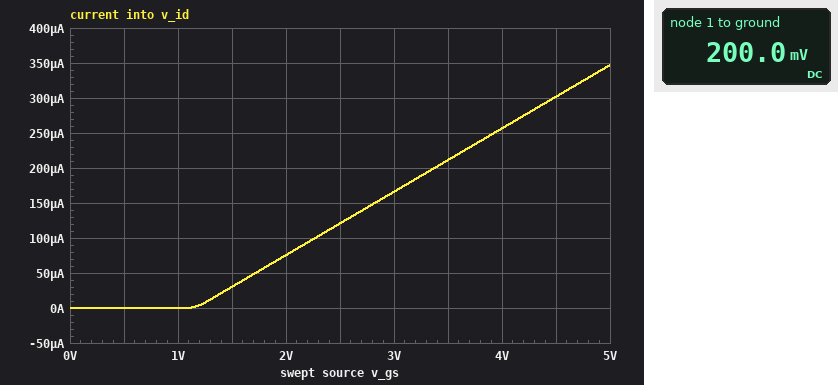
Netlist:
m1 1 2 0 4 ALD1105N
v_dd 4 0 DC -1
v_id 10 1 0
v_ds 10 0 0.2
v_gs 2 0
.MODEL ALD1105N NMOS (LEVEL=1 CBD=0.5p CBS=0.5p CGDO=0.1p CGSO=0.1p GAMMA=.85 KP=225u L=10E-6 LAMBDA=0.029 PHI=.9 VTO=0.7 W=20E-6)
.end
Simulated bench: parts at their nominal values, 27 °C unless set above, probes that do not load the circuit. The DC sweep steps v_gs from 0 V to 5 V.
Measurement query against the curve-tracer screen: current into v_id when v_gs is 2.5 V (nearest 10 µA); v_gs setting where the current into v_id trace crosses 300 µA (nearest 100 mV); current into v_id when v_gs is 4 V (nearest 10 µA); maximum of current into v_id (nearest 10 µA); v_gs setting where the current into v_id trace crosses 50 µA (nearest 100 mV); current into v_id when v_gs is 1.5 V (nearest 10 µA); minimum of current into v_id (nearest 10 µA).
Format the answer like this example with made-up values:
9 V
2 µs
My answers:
120 µA
4.5 V
260 µA
350 µA
1.7 V
30 µA
0 A
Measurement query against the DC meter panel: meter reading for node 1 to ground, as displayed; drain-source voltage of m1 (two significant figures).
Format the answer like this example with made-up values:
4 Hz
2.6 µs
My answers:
200.0 mV
200 mV
